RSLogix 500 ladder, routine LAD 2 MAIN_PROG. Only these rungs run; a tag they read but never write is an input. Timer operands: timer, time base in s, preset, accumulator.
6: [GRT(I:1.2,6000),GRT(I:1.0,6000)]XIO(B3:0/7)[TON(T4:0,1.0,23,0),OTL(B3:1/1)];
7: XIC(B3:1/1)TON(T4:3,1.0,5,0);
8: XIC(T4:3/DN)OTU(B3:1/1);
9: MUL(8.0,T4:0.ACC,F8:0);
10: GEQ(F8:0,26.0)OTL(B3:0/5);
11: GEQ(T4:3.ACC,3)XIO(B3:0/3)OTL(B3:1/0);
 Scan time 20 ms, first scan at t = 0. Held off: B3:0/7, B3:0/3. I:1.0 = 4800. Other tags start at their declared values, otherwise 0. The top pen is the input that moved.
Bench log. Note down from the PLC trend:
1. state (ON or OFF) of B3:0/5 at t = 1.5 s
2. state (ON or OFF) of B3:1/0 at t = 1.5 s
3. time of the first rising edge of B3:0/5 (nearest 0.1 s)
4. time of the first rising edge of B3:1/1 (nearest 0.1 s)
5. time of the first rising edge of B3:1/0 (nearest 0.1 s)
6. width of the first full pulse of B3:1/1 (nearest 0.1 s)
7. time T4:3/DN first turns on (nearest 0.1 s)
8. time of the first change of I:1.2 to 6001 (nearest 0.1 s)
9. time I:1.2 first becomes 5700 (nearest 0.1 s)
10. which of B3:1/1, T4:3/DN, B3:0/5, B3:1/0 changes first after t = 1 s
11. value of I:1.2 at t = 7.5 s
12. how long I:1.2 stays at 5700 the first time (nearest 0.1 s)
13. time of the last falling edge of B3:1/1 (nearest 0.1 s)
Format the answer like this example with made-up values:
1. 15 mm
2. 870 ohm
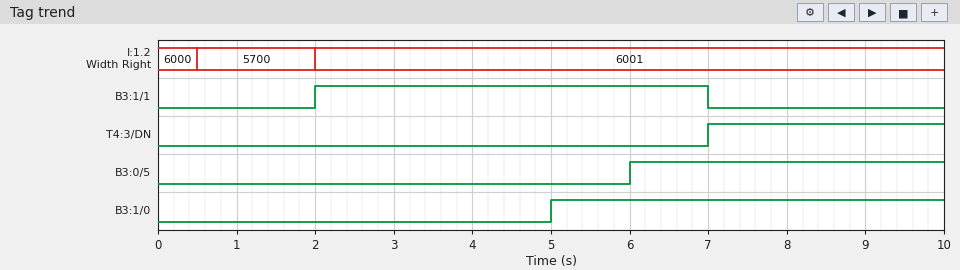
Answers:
1. OFF
2. OFF
3. 6.0 s
4. 2.0 s
5. 5.0 s
6. 5.0 s
7. 7.0 s
8. 2.0 s
9. 0.5 s
10. B3:1/1
11. 6001
12. 1.5 s
13. 7.0 s
